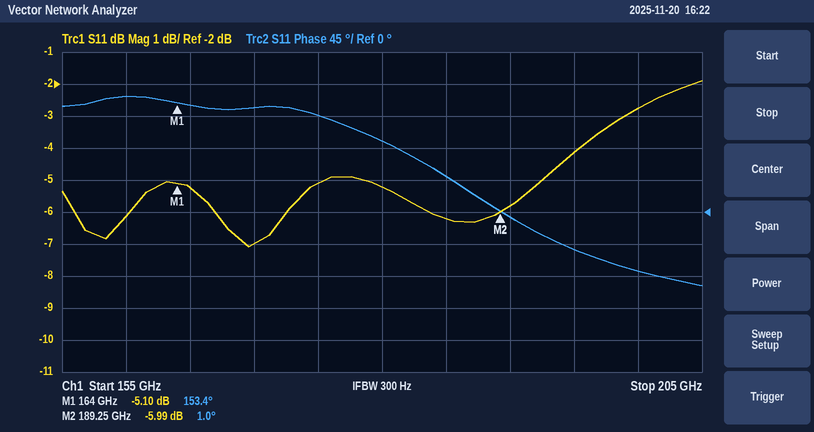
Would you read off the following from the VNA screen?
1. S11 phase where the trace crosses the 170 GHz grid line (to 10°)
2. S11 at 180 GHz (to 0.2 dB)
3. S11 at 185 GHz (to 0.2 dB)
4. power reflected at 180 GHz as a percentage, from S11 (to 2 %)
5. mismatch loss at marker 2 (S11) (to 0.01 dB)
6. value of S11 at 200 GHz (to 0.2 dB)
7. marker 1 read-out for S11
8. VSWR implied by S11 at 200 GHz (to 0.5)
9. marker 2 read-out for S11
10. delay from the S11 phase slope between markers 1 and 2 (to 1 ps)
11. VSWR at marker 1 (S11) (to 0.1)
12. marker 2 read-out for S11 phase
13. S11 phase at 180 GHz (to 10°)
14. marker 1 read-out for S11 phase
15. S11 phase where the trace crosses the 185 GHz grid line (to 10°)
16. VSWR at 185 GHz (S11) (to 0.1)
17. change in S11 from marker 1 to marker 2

150°
-5.2 dB
-6.2 dB
30 %
1.26 dB
-2.8 dB
-5.10 dB
6.5
-5.99 dB
17 ps
3.5
1.0°
100°
153.4°
50°
2.9
-0.89 dB
